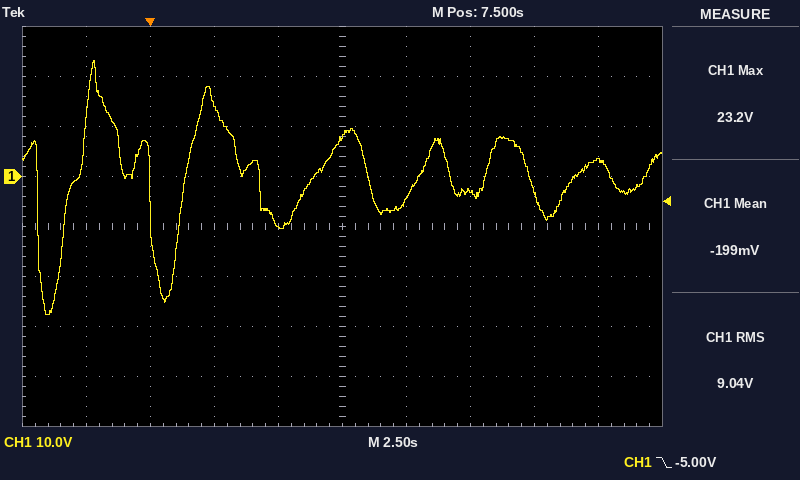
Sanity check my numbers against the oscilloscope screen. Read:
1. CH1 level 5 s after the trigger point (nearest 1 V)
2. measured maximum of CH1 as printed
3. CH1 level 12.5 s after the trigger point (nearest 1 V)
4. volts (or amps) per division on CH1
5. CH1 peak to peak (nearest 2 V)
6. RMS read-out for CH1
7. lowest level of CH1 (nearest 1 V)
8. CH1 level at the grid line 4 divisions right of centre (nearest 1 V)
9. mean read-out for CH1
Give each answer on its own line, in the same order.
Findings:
-10 V
23.2 V
-3 V
10 V
50 V
9.04 V
-28 V
3 V
-199 mV
